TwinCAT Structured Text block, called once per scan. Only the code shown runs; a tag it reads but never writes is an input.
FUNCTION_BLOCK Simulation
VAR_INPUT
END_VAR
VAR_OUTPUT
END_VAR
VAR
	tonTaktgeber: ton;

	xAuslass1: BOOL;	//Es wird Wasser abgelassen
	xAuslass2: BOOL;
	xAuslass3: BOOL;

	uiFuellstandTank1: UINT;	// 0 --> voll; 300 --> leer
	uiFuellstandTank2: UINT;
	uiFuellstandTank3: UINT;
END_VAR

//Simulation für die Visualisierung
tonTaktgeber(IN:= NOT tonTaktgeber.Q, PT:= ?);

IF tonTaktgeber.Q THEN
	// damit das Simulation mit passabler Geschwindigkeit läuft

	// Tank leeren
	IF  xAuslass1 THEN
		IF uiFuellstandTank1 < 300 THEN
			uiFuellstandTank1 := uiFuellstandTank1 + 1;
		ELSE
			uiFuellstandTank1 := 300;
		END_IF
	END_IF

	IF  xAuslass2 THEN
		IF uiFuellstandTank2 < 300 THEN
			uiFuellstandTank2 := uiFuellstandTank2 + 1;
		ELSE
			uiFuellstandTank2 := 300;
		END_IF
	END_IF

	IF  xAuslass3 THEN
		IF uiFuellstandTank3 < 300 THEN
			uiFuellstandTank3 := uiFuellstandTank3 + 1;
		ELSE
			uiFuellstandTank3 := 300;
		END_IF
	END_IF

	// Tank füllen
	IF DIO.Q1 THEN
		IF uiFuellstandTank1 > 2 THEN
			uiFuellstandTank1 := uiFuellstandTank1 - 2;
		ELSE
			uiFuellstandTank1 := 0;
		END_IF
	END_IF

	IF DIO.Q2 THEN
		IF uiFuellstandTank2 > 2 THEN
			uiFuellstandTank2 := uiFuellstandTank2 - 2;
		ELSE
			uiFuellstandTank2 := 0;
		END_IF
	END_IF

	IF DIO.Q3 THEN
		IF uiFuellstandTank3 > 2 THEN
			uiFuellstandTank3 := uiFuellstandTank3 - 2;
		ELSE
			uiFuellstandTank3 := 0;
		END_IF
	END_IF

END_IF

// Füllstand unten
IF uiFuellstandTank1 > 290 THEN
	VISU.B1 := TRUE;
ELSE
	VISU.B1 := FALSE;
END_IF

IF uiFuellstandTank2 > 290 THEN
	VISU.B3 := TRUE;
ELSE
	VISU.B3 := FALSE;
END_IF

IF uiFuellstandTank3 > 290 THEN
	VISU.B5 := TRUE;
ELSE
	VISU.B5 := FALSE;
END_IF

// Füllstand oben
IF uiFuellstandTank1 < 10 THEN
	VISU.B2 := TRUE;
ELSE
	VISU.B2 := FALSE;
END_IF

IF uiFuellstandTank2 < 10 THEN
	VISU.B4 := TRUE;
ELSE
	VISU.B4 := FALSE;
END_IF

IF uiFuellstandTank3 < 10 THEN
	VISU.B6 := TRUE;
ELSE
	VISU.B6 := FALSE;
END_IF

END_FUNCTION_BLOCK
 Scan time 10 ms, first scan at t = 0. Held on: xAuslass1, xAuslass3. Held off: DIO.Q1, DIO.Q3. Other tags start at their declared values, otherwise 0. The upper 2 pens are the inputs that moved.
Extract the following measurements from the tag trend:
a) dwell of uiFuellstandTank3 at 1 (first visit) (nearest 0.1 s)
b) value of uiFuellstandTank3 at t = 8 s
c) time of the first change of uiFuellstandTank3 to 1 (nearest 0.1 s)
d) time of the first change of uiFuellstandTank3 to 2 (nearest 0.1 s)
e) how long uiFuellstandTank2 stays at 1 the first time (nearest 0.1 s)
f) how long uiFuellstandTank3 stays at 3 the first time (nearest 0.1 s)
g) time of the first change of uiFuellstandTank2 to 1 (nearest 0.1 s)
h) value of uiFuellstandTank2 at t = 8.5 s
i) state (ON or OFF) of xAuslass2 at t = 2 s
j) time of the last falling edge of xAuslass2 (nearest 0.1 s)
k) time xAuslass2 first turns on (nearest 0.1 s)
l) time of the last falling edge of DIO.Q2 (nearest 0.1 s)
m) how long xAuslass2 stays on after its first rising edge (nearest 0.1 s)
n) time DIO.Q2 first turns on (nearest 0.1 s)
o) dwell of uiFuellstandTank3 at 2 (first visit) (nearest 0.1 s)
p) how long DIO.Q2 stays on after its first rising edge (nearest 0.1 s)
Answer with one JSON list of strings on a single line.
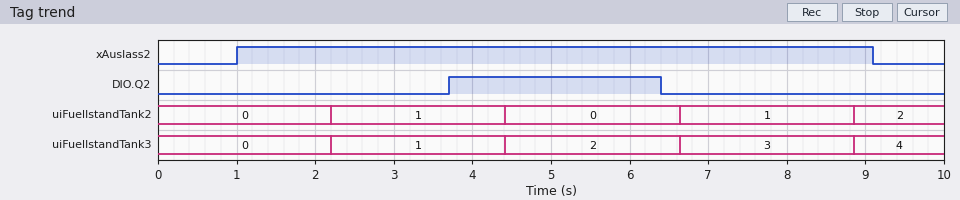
["2.2 s", "3", "2.2 s", "4.4 s", "2.2 s", "2.2 s", "2.2 s", "1", "ON", "9.1 s", "1.0 s", "6.4 s", "8.1 s", "3.7 s", "2.2 s", "2.7 s"]
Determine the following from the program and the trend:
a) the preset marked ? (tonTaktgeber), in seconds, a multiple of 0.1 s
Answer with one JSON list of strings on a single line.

["2.2 s"]
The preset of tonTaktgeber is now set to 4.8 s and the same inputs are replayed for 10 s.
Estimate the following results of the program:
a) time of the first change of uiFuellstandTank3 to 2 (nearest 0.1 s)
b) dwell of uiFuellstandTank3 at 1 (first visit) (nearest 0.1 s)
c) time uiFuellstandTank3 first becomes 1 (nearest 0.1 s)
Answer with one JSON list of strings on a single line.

["9.6 s", "4.8 s", "4.8 s"]
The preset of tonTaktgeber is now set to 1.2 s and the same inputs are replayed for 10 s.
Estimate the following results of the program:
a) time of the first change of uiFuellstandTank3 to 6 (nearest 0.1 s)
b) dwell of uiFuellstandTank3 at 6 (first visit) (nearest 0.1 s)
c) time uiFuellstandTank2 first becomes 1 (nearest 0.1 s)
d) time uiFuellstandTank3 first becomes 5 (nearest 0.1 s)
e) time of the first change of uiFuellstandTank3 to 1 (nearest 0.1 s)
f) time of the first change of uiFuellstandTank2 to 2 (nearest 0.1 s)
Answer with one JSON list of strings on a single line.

["7.3 s", "1.2 s", "1.2 s", "6.1 s", "1.2 s", "2.4 s"]
